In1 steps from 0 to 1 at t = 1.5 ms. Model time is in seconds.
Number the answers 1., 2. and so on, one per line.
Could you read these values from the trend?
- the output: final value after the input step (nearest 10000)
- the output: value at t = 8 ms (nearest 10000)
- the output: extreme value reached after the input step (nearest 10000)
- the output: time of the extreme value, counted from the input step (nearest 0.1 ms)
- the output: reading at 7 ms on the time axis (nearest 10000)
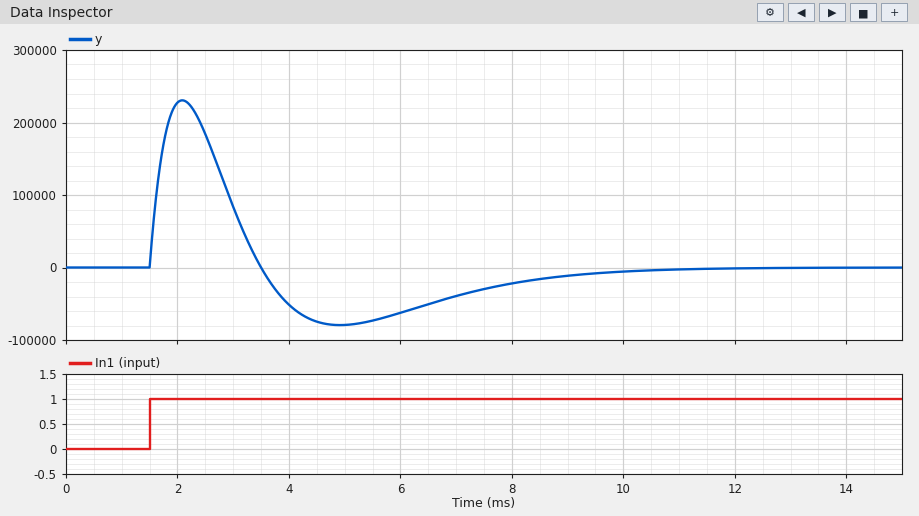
1. 0
2. -20000
3. 230000
4. 0.6 ms
5. -40000
